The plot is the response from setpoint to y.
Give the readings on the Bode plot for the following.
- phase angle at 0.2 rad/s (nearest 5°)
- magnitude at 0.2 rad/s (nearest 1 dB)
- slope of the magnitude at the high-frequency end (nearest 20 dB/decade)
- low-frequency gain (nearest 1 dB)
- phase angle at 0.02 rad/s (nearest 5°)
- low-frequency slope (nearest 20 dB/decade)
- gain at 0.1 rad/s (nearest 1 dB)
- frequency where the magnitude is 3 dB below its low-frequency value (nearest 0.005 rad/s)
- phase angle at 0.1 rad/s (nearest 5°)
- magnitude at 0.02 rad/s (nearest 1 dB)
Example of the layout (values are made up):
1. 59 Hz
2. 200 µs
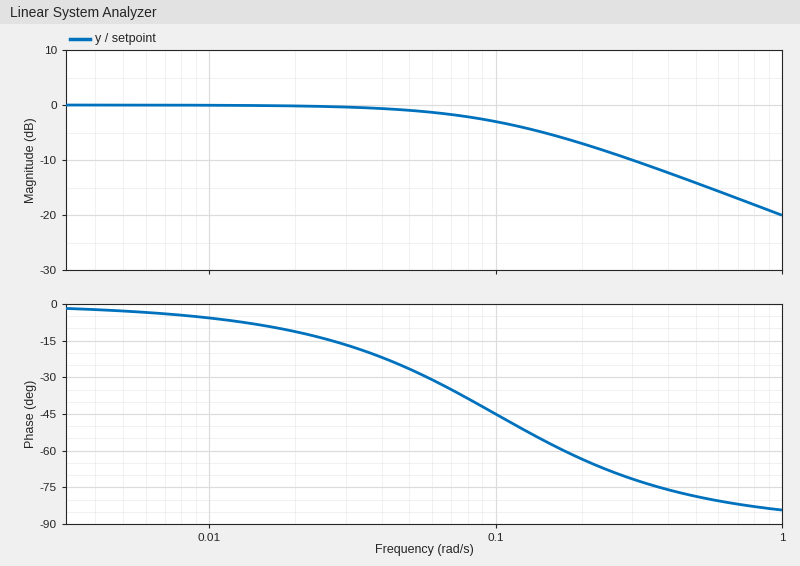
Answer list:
1. -65°
2. -7 dB
3. -20 dB/decade
4. 0 dB
5. -10°
6. 0 dB/decade
7. -3 dB
8. 0.100 rad/s
9. -45°
10. 0 dB
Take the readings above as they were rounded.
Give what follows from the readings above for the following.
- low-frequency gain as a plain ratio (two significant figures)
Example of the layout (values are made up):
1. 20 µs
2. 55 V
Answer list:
1. 1.0
